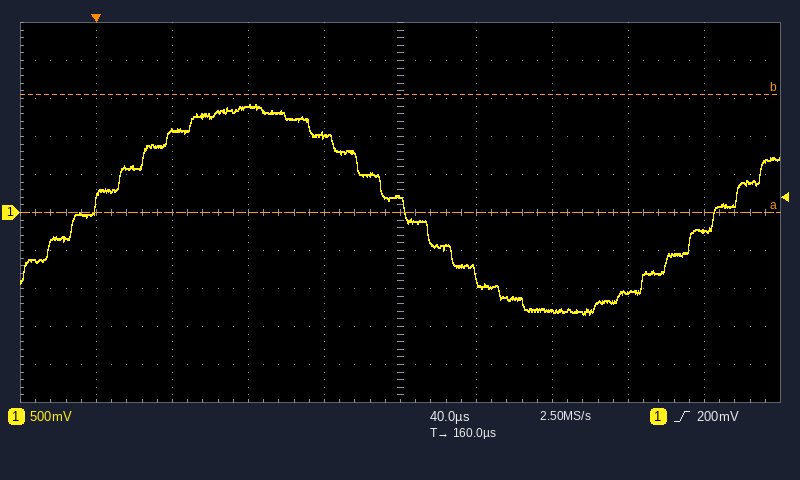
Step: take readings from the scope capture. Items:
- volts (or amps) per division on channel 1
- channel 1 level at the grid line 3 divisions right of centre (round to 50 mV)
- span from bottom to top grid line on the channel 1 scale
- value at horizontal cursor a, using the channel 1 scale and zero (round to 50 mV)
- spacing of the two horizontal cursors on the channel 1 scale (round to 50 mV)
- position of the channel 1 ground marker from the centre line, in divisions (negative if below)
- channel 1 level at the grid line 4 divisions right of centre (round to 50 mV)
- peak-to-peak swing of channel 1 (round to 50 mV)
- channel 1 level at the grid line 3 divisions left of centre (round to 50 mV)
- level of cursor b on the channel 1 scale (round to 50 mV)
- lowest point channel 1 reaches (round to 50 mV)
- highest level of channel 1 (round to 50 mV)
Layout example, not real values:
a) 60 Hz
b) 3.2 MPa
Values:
a) 500 mV
b) -1.05 V
c) 5 V
d) 0 mV
e) 1.55 V
f) 0.0 div
g) -250 mV
h) 2.75 V
i) 1.05 V
j) 1.55 V
k) -1.35 V
l) 1.40 V
